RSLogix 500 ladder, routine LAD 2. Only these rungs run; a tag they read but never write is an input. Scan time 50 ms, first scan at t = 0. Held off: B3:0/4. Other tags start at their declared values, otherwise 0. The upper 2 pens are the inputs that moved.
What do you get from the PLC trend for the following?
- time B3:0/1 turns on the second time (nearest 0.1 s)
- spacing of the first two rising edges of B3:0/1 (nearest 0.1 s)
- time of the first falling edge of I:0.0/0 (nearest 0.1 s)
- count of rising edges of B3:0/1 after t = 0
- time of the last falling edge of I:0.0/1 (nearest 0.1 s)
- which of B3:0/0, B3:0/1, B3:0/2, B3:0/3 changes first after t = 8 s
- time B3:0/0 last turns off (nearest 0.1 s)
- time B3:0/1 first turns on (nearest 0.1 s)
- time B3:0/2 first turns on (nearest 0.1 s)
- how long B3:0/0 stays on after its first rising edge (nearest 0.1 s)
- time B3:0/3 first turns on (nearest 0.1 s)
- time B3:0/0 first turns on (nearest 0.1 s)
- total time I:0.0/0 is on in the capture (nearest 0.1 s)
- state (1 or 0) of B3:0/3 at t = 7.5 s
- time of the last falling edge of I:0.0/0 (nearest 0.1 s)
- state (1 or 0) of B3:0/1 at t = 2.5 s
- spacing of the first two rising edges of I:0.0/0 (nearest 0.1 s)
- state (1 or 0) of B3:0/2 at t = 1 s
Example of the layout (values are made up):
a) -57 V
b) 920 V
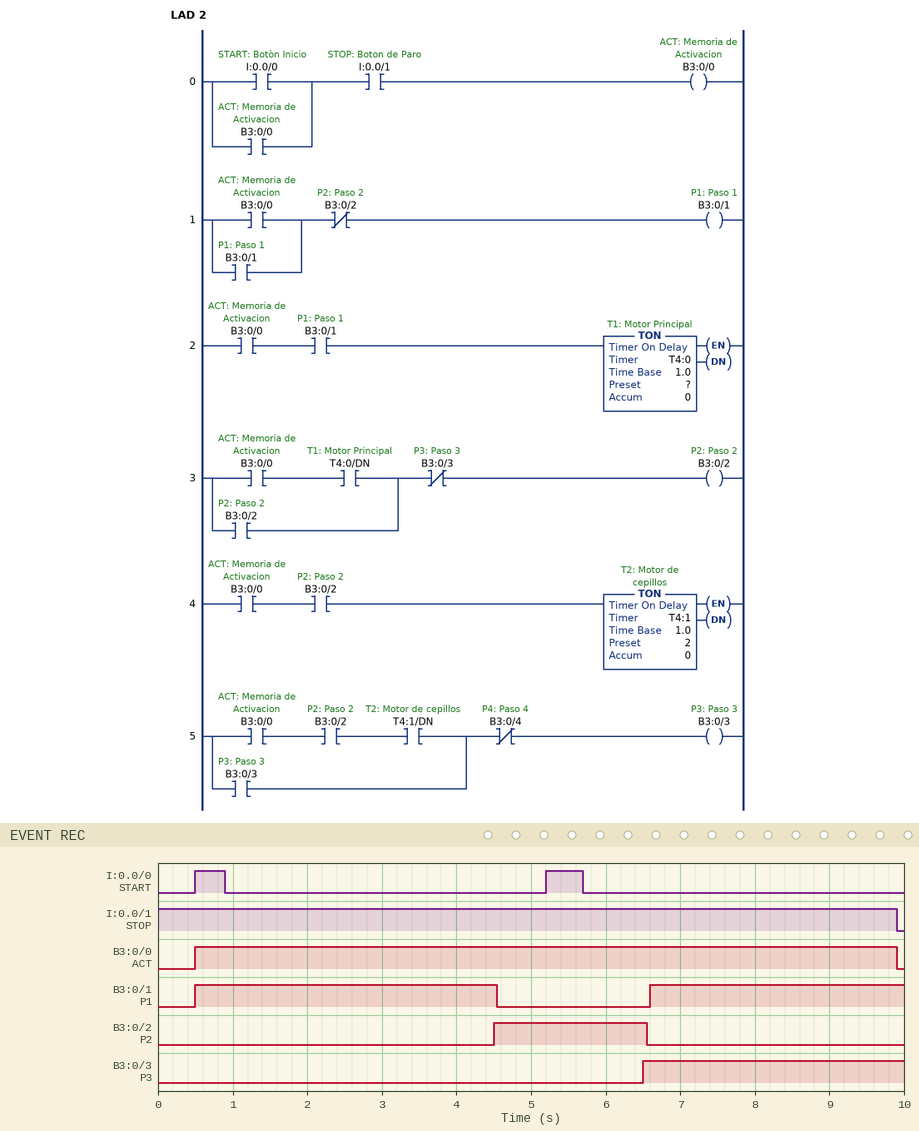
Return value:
a) 6.6 s
b) 6.1 s
c) 0.9 s
d) 2
e) 9.9 s
f) B3:0/0
g) 9.9 s
h) 0.5 s
i) 4.5 s
j) 9.4 s
k) 6.5 s
l) 0.5 s
m) 0.9 s
n) 1
o) 5.7 s
p) 1
q) 4.7 s
r) 0
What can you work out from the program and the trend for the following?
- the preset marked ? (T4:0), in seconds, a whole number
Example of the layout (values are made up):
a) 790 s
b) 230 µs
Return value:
a) 4 s
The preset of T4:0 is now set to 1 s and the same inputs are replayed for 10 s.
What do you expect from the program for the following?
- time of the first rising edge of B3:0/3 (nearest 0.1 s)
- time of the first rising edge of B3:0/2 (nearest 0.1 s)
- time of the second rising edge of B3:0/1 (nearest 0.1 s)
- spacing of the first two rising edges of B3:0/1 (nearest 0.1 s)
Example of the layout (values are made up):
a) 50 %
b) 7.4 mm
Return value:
a) 3.5 s
b) 1.5 s
c) 3.6 s
d) 3.1 s
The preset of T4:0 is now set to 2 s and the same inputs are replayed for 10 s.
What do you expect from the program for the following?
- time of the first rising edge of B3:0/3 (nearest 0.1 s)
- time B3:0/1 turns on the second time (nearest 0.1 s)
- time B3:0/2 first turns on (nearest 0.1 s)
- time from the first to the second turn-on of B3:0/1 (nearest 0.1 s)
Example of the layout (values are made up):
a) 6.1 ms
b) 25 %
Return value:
a) 4.5 s
b) 4.6 s
c) 2.5 s
d) 4.1 s
